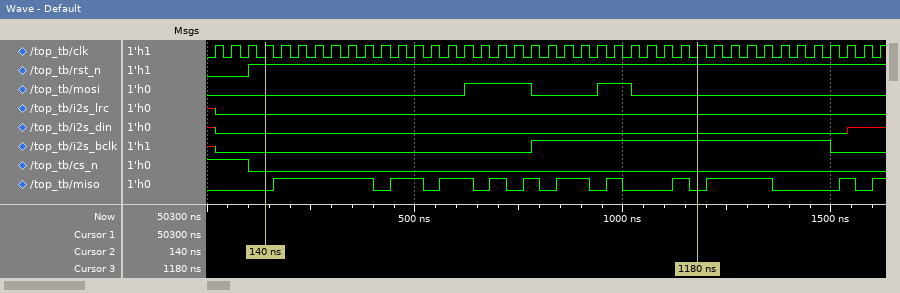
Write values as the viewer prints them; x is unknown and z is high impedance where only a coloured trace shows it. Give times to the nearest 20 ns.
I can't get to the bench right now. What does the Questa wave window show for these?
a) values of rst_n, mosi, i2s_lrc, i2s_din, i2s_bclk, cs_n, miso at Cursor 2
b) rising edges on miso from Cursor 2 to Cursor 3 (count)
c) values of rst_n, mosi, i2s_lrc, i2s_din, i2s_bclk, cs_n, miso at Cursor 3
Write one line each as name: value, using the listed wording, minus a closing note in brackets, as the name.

values of rst_n, mosi, i2s_lrc, i2s_din, i2s_bclk, cs_n, miso at Cursor 2: rst_n=1, mosi=0, i2s_lrc=0, i2s_din=0, i2s_bclk=0, cs_n=0, miso=0
rising edges on miso from Cursor 2 to Cursor 3: 8
values of rst_n, mosi, i2s_lrc, i2s_din, i2s_bclk, cs_n, miso at Cursor 3: rst_n=1, mosi=0, i2s_lrc=0, i2s_din=0, i2s_bclk=1, cs_n=0, miso=0
